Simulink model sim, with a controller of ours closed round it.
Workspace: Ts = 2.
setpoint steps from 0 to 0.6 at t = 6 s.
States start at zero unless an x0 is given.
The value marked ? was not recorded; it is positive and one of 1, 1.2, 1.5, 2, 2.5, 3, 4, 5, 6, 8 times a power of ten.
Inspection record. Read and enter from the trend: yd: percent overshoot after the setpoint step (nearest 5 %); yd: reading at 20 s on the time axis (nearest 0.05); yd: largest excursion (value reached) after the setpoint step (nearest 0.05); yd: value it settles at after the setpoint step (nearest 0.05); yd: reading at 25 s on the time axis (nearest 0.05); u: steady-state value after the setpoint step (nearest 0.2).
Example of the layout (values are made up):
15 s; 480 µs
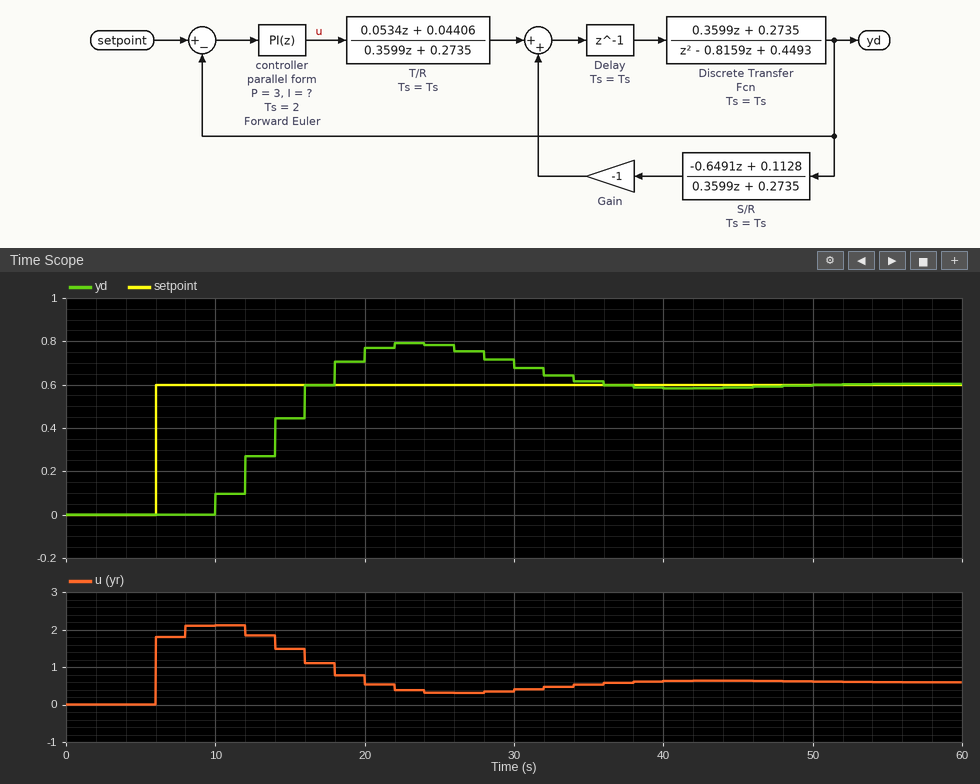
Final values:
30 %; 0.75; 0.80; 0.60; 0.80; 0.6
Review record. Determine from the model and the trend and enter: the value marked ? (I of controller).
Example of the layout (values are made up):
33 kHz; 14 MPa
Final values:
0.25
